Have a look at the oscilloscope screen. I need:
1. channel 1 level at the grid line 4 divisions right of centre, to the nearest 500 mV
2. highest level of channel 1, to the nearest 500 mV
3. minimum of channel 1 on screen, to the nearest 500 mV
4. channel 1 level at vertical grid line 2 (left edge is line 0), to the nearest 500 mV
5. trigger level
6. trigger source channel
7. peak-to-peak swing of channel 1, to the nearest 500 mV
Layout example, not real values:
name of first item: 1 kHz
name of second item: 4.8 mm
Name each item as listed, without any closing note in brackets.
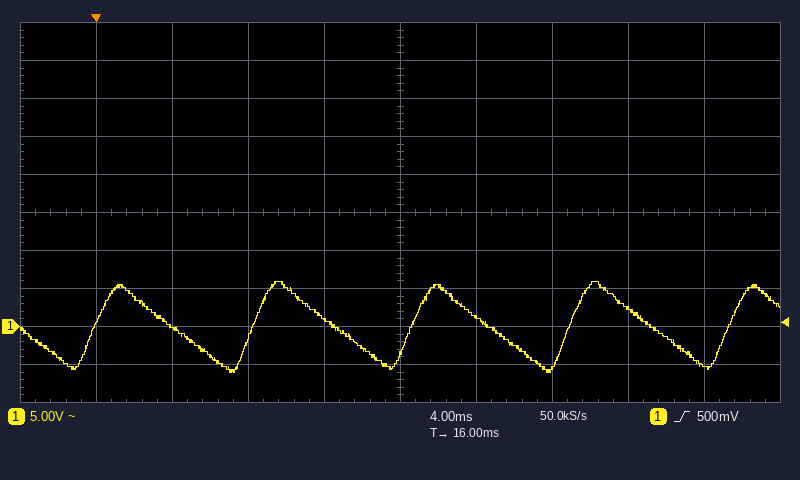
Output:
channel 1 level at the grid line 4 divisions right of centre, to the nearest 500 mV: -5.5 V
highest level of channel 1, to the nearest 500 mV: 6.0 V
minimum of channel 1 on screen, to the nearest 500 mV: -6.0 V
channel 1 level at vertical grid line 2 (left edge is line 0), to the nearest 500 mV: 0.0 V
trigger level: 500 mV
trigger source channel: channel 1
peak-to-peak swing of channel 1, to the nearest 500 mV: 12.0 V
